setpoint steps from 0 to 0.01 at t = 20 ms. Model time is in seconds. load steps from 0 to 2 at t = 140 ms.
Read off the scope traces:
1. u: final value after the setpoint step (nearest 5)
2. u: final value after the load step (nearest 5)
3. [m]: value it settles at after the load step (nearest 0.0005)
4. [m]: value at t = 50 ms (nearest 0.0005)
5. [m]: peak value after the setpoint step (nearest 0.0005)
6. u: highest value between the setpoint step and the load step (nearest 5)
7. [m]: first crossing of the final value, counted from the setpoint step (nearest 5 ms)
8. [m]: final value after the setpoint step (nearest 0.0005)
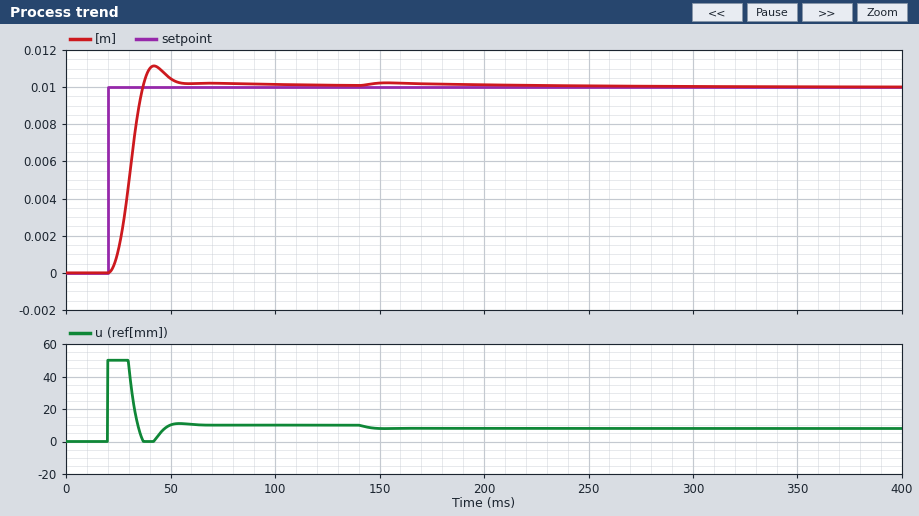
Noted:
10
10
0.0100
0.0105
0.0110
50
15 ms
0.0100
